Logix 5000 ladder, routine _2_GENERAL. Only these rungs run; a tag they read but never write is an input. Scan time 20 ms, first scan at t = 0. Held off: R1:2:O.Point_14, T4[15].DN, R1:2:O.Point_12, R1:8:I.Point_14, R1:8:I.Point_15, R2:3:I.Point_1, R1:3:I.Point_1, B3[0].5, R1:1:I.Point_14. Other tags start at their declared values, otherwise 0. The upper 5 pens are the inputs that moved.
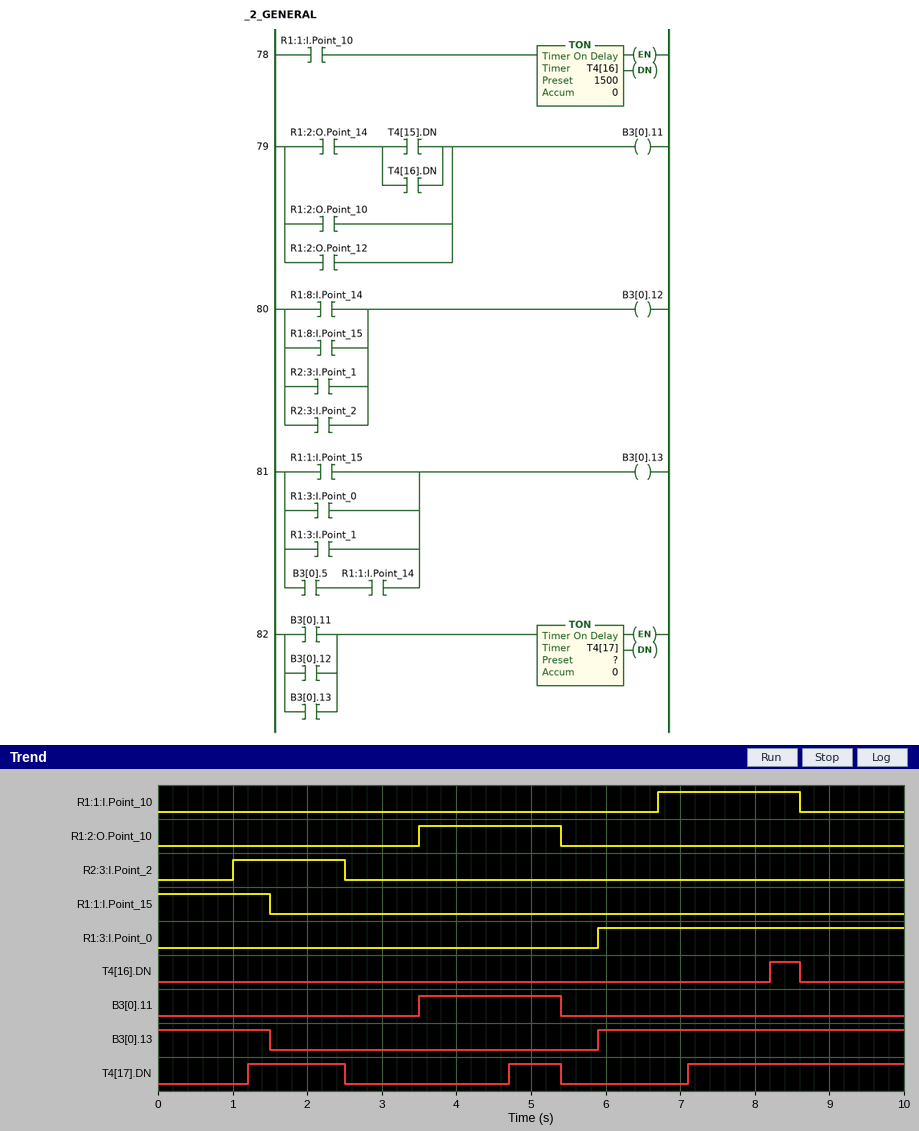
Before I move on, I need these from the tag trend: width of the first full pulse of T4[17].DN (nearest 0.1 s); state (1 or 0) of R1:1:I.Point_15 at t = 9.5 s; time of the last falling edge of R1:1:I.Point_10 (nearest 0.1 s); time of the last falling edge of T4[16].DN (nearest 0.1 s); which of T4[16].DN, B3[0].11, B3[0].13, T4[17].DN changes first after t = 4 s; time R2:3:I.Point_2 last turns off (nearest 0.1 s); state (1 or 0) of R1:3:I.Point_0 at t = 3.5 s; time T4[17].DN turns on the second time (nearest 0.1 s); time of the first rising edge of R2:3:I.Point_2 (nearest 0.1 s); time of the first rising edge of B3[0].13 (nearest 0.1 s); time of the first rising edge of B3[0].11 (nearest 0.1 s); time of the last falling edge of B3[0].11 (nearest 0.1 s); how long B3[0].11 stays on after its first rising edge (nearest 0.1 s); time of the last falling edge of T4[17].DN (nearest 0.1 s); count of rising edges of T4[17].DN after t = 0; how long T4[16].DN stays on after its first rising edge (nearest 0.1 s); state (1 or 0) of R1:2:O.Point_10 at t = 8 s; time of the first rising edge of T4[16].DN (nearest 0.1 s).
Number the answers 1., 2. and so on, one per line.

1. 1.3 s
2. 0
3. 8.6 s
4. 8.6 s
5. T4[17].DN
6. 2.5 s
7. 0
8. 4.7 s
9. 1.0 s
10. 5.9 s
11. 3.5 s
12. 5.4 s
13. 1.9 s
14. 5.4 s
15. 3
16. 0.4 s
17. 0
18. 8.2 s
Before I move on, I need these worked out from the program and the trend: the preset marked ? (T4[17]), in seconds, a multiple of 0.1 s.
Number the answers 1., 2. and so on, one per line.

1. 1.2 s
